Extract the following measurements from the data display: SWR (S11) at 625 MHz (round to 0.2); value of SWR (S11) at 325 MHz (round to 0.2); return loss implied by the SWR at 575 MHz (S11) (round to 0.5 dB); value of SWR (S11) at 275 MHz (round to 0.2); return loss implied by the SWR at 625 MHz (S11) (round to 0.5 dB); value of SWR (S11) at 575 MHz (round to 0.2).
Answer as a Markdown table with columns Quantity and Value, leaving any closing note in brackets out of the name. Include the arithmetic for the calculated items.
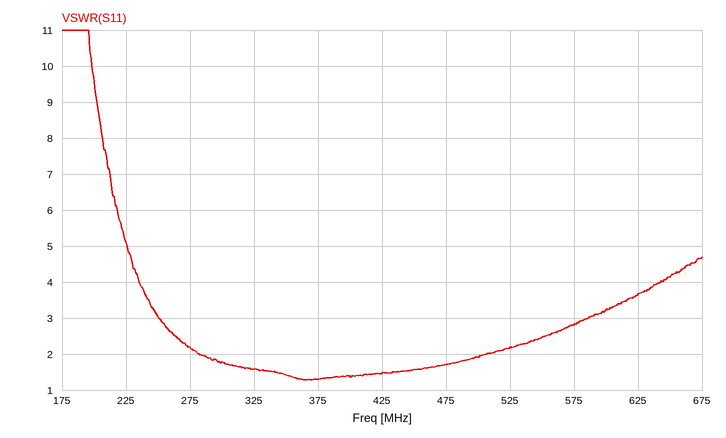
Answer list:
| Quantity | Value |
|---|---|
| SWR (S11) at 625 MHz | 3.6 |
| value of SWR (S11) at 325 MHz | 1.6 |
| return loss implied by the SWR at 575 MHz (S11) | −20 log10((2.8 − 1)/(2.8 + 1)) ≈ 6.5 dB |
| value of SWR (S11) at 275 MHz | 2.2 |
| return loss implied by the SWR at 625 MHz (S11) | −20 log10((3.6 − 1)/(3.6 + 1)) ≈ 5.0 dB |
| value of SWR (S11) at 575 MHz | 2.8 |
